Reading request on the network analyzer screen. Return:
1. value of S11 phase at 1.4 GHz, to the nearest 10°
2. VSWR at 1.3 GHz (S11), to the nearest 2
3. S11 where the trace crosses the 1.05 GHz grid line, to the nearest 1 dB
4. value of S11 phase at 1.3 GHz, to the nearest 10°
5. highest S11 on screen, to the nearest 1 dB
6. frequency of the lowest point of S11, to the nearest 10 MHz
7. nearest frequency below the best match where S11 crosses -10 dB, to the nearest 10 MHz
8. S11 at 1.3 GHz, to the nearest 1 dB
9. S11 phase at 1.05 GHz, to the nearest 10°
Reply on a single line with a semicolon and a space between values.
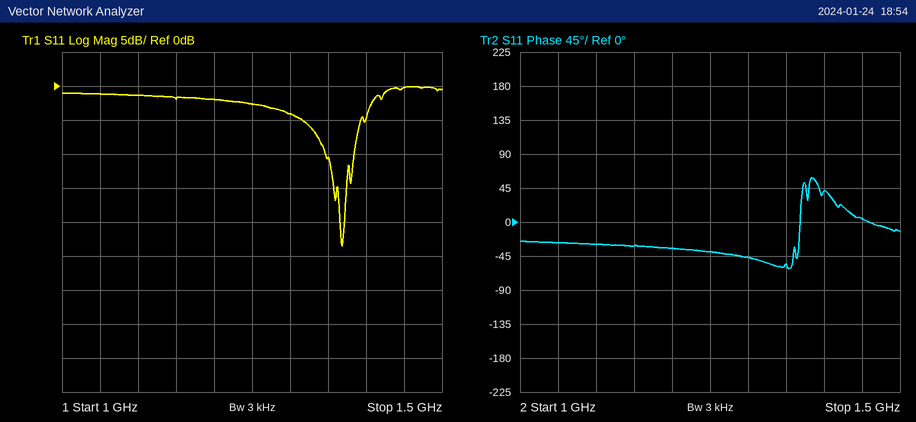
40°; 4; -1 dB; -50°; 0 dB; 1.37 GHz; 1.35 GHz; -4 dB; -30°
